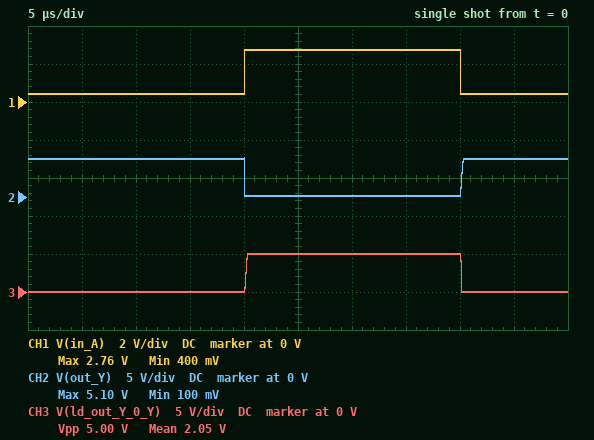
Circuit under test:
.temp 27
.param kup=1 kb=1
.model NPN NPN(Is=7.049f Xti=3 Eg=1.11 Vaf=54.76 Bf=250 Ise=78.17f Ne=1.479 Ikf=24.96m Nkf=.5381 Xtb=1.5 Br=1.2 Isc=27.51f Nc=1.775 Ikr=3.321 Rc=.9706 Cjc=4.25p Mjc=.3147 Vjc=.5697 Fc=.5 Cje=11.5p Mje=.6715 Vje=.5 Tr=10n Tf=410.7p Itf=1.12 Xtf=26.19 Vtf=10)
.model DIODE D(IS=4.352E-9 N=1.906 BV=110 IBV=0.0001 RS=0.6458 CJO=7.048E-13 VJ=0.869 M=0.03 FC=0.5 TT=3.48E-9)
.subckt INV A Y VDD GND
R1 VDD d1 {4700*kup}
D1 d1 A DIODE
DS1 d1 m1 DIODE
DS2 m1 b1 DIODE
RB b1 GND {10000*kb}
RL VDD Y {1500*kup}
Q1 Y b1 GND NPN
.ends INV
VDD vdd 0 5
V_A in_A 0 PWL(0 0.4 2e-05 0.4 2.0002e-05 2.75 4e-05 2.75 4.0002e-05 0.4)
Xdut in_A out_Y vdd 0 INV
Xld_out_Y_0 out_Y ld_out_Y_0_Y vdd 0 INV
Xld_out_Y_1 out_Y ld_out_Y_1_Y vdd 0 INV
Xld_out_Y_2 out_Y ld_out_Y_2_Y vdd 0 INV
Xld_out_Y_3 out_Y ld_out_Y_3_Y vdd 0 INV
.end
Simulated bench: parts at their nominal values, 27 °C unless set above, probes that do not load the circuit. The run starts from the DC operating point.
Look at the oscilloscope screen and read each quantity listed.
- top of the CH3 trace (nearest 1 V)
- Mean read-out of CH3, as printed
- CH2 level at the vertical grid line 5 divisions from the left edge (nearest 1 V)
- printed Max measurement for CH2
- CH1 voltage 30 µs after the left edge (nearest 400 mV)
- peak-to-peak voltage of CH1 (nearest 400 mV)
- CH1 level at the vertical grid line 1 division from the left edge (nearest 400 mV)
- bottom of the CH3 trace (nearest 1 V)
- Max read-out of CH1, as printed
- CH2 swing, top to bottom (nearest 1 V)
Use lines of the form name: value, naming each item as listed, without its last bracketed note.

top of the CH3 trace: 5 V
Mean read-out of CH3, as printed: 2.05 V
CH2 level at the vertical grid line 5 divisions from the left edge: 0 V
printed Max measurement for CH2: 5.10 V
CH1 voltage 30 µs after the left edge: 2.8 V
peak-to-peak voltage of CH1: 2.4 V
CH1 level at the vertical grid line 1 division from the left edge: 400 mV
bottom of the CH3 trace: 0 V
Max read-out of CH1, as printed: 2.76 V
CH2 swing, top to bottom: 5 V
